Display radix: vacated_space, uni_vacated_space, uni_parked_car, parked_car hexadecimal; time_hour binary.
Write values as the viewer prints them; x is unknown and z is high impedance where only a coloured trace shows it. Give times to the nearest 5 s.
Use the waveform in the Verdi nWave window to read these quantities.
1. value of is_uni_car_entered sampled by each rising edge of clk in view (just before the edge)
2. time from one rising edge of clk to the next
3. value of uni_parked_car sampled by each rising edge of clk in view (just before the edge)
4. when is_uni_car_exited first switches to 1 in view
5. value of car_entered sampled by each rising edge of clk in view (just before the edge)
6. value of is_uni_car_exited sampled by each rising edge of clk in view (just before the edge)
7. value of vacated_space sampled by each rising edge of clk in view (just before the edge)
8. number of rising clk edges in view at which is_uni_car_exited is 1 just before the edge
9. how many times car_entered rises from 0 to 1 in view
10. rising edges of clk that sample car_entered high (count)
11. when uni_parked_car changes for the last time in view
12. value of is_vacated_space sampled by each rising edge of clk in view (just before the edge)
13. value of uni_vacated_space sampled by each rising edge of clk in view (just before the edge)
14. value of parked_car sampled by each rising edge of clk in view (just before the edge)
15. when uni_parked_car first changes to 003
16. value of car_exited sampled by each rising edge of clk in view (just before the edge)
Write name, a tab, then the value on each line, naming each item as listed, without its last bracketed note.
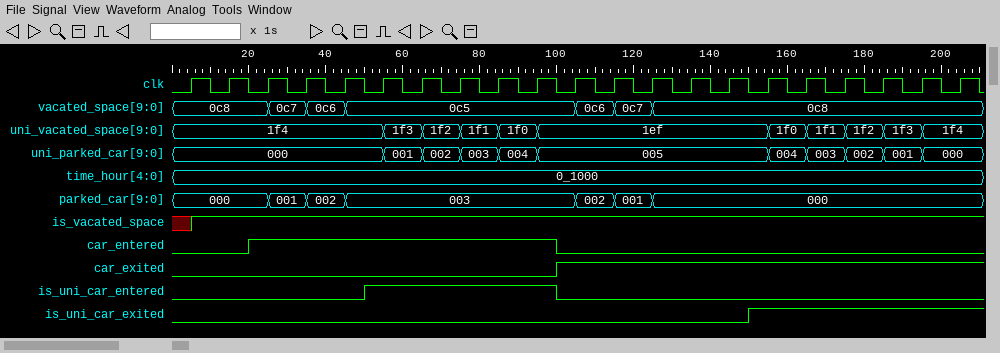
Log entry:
value of is_uni_car_entered sampled by each rising edge of clk in view	0 0 0 0 0 1 1 1 1 1 0 0 0 0 0 0 0 0 0 0 0
time from one rising edge of clk to the next	10 s
value of uni_parked_car sampled by each rising edge of clk in view	000, 000, 000, 000, 000, 000, 001, 002, 003, 004, 005, 005, 005, 005, 005, 005, 004, 003, 002, 001, 000
when is_uni_car_exited first switches to 1 in view	150 s
value of car_entered sampled by each rising edge of clk in view	0 0 1 1 1 1 1 1 1 1 0 0 0 0 0 0 0 0 0 0 0
value of is_uni_car_exited sampled by each rising edge of clk in view	0 0 0 0 0 0 0 0 0 0 0 0 0 0 0 1 1 1 1 1 1
value of vacated_space sampled by each rising edge of clk in view	0c8, 0c8, 0c8, 0c7, 0c6, 0c5, 0c5, 0c5, 0c5, 0c5, 0c5, 0c6, 0c7, 0c8, 0c8, 0c8, 0c8, 0c8, 0c8, 0c8, 0c8
number of rising clk edges in view at which is_uni_car_exited is 1 just before the edge	6
how many times car_entered rises from 0 to 1 in view	1
rising edges of clk that sample car_entered high	8
when uni_parked_car changes for the last time in view	195 s
value of is_vacated_space sampled by each rising edge of clk in view	x 1 1 1 1 1 1 1 1 1 1 1 1 1 1 1 1 1 1 1 1
value of uni_vacated_space sampled by each rising edge of clk in view	1f4, 1f4, 1f4, 1f4, 1f4, 1f4, 1f3, 1f2, 1f1, 1f0, 1ef, 1ef, 1ef, 1ef, 1ef, 1ef, 1f0, 1f1, 1f2, 1f3, 1f4
value of parked_car sampled by each rising edge of clk in view	000, 000, 000, 001, 002, 003, 003, 003, 003, 003, 003, 002, 001, 000, 000, 000, 000, 000, 000, 000, 000
when uni_parked_car first changes to 003	75 s
value of car_exited sampled by each rising edge of clk in view	0 0 0 0 0 0 0 0 0 0 1 1 1 1 1 1 1 1 1 1 1
